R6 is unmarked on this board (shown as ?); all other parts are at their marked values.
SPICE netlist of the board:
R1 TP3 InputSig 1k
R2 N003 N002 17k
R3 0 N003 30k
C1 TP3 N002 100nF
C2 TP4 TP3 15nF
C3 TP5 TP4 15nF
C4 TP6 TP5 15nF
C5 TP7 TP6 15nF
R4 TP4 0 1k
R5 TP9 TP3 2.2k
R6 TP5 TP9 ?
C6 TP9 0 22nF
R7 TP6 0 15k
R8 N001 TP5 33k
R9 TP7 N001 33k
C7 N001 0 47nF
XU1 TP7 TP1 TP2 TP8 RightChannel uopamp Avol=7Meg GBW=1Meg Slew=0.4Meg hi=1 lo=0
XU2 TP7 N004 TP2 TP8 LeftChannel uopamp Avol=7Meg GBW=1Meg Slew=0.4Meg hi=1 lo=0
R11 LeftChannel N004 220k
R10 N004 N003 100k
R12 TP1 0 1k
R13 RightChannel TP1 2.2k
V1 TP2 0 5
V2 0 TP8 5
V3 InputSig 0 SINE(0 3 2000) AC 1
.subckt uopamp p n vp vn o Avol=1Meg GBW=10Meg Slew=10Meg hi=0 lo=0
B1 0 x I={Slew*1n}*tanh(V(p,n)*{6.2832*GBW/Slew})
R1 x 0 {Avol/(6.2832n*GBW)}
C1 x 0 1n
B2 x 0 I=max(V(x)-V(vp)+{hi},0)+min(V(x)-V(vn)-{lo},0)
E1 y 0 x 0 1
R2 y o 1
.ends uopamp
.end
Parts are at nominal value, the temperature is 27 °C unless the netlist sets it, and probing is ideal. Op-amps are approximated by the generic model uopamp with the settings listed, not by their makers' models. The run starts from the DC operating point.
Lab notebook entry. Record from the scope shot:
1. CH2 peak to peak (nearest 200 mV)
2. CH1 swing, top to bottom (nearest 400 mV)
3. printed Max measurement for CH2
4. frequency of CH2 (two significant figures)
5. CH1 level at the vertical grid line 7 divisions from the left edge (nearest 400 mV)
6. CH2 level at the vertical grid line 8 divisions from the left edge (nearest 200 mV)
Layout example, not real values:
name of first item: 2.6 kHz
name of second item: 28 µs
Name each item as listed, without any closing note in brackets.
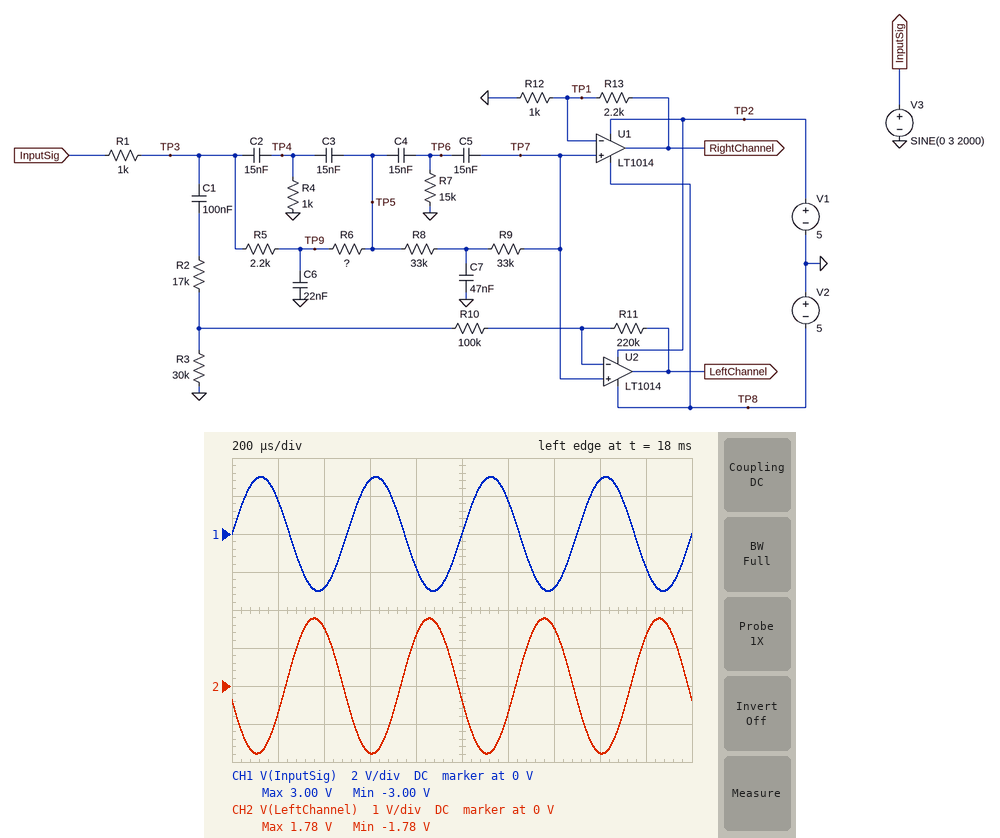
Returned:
CH2 peak to peak: 3.6 V
CH1 swing, top to bottom: 6.0 V
printed Max measurement for CH2: 1.78 V
frequency of CH2: 2.0 kHz
CH1 level at the vertical grid line 7 divisions from the left edge: -2.8 V
CH2 level at the vertical grid line 8 divisions from the left edge: -1.8 V
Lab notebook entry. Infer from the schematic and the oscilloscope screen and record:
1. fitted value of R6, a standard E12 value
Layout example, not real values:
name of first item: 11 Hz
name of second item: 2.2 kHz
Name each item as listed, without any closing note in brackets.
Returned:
fitted value of R6, a standard E12 value: 4.7 kΩ
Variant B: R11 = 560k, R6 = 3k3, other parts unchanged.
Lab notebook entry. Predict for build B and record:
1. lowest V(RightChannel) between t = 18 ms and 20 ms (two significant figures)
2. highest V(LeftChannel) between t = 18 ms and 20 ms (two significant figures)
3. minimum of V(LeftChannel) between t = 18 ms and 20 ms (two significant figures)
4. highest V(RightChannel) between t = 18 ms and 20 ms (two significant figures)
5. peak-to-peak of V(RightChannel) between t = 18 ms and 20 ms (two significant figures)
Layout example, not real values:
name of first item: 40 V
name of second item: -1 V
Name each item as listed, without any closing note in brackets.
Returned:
lowest V(RightChannel) between t = 18 ms and 20 ms: -2.0 V
highest V(LeftChannel) between t = 18 ms and 20 ms: 4.0 V
minimum of V(LeftChannel) between t = 18 ms and 20 ms: -4.2 V
highest V(RightChannel) between t = 18 ms and 20 ms: 2.0 V
peak-to-peak of V(RightChannel) between t = 18 ms and 20 ms: 4.1 V
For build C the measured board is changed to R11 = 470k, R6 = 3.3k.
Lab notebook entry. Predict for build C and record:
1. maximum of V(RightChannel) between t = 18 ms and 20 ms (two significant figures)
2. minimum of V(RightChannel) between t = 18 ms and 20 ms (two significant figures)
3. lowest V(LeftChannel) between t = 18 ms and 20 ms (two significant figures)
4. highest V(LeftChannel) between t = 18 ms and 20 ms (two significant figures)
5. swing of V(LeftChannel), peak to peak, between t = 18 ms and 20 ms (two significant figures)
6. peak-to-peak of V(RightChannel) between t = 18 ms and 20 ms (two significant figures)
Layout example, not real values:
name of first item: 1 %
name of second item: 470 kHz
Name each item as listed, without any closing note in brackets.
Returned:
maximum of V(RightChannel) between t = 18 ms and 20 ms: 2.0 V
minimum of V(RightChannel) between t = 18 ms and 20 ms: -2.0 V
lowest V(LeftChannel) between t = 18 ms and 20 ms: -3.5 V
highest V(LeftChannel) between t = 18 ms and 20 ms: 3.5 V
swing of V(LeftChannel), peak to peak, between t = 18 ms and 20 ms: 7.0 V
peak-to-peak of V(RightChannel) between t = 18 ms and 20 ms: 4.1 V
